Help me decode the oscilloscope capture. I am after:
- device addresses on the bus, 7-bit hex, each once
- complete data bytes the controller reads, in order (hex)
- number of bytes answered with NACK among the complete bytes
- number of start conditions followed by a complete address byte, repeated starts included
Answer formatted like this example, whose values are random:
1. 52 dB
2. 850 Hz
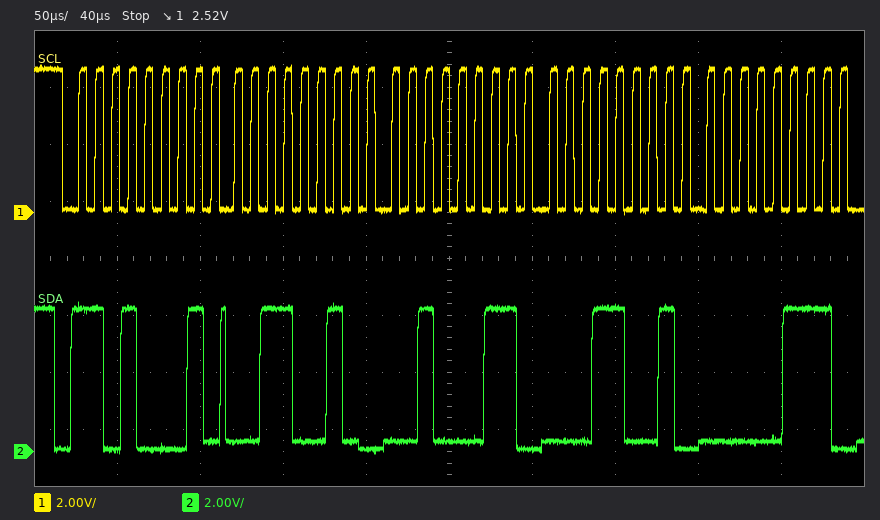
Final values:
1. 0x68
2. 32 23 19 07
3. 0
4. 1
